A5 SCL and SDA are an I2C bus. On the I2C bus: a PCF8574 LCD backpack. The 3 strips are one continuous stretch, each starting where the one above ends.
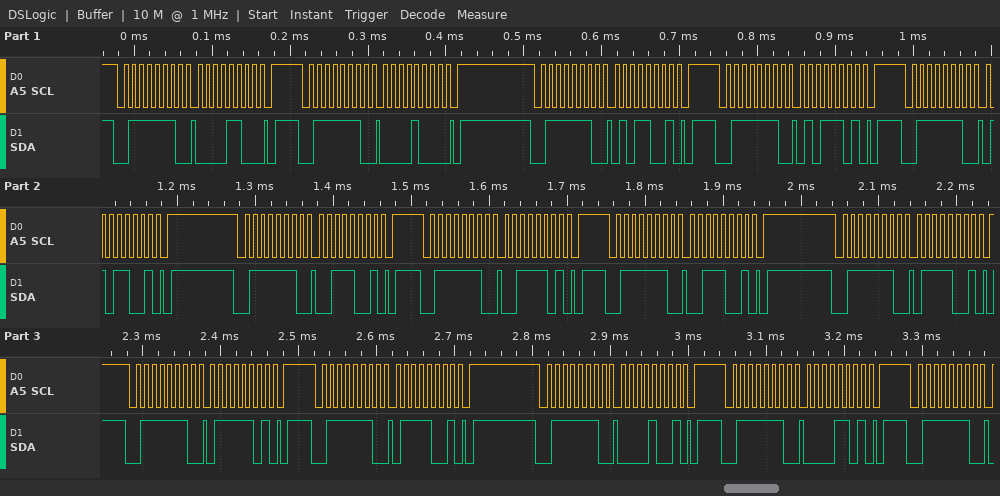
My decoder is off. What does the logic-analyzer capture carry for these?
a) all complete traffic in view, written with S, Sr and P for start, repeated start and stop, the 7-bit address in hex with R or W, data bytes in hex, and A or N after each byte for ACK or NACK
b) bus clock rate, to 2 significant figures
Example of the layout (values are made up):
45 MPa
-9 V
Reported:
S 3FW A 0C A P S 3FW A 08 A P S 3FW A 59 A P S 3FW A 5D A P S 3FW A 59 A P S 3FW A 39 A P S 3FW A 3D A P S 3FW A 39 A P S 3FW A 79 A P S 3FW A 7D A P S 3FW A 79 A P S 3FW A 09 A P S 3FW A 0D A P S 3FW A
100 kHz
